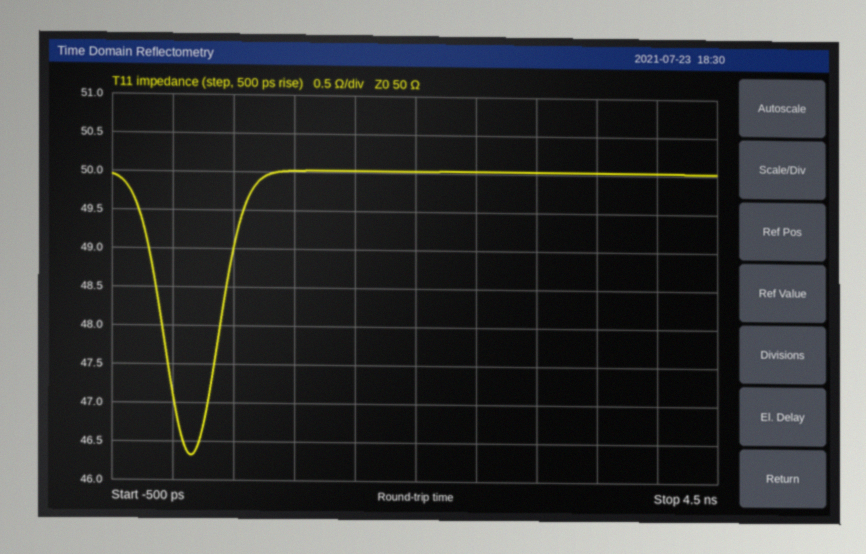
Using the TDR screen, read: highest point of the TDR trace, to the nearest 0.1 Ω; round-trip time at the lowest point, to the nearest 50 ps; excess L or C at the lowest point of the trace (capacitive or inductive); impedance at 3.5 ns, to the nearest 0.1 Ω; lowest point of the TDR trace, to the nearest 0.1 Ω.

50.0 Ω
150 ps
capacitive
50.0 Ω
46.3 Ω
